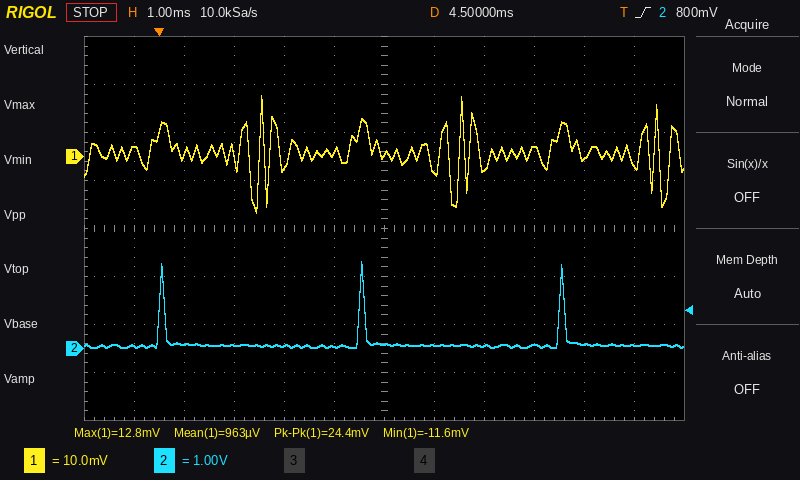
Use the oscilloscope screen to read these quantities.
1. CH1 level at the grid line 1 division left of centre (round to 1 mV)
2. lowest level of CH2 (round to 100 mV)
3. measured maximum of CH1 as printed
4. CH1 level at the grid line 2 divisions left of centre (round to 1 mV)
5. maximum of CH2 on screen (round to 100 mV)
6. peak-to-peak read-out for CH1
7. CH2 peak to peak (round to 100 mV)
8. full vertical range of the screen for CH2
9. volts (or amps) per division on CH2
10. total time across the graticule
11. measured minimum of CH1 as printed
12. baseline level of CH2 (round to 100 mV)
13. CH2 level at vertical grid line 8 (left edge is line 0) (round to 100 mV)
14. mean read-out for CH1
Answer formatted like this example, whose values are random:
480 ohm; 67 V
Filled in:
1 mV; 0.0 V; 12.8 mV; -2 mV; 1.8 V; 24.4 mV; 1.8 V; 8 V; 1 V; 12 ms; -11.6 mV; 100 mV; 100 mV; 963 µV
